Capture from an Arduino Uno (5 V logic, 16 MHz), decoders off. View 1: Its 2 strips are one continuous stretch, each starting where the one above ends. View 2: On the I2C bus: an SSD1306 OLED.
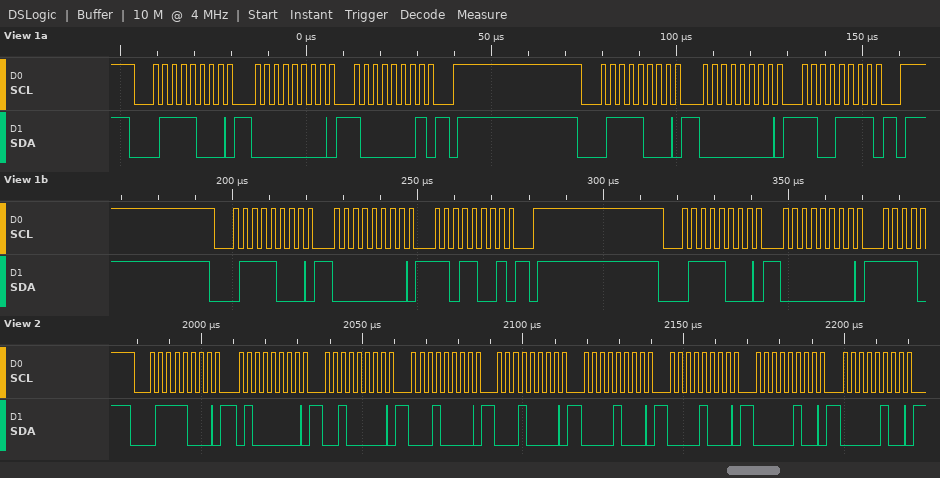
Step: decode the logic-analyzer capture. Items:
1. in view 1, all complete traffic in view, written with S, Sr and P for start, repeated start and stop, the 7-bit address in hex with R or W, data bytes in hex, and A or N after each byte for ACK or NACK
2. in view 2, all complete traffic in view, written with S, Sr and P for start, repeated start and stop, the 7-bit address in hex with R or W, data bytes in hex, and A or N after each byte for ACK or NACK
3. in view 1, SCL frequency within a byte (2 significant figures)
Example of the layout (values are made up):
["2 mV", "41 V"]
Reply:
["S 3CW A 00 A 81 A P S 3CW A 00 A CF A P S 3CW A 00 A D9 A P S 3CW A 00 A", "S 3CW A 40 A 20 A 10 A 10 A 08 A 08 A 04 A 04 A", "400 kHz"]
